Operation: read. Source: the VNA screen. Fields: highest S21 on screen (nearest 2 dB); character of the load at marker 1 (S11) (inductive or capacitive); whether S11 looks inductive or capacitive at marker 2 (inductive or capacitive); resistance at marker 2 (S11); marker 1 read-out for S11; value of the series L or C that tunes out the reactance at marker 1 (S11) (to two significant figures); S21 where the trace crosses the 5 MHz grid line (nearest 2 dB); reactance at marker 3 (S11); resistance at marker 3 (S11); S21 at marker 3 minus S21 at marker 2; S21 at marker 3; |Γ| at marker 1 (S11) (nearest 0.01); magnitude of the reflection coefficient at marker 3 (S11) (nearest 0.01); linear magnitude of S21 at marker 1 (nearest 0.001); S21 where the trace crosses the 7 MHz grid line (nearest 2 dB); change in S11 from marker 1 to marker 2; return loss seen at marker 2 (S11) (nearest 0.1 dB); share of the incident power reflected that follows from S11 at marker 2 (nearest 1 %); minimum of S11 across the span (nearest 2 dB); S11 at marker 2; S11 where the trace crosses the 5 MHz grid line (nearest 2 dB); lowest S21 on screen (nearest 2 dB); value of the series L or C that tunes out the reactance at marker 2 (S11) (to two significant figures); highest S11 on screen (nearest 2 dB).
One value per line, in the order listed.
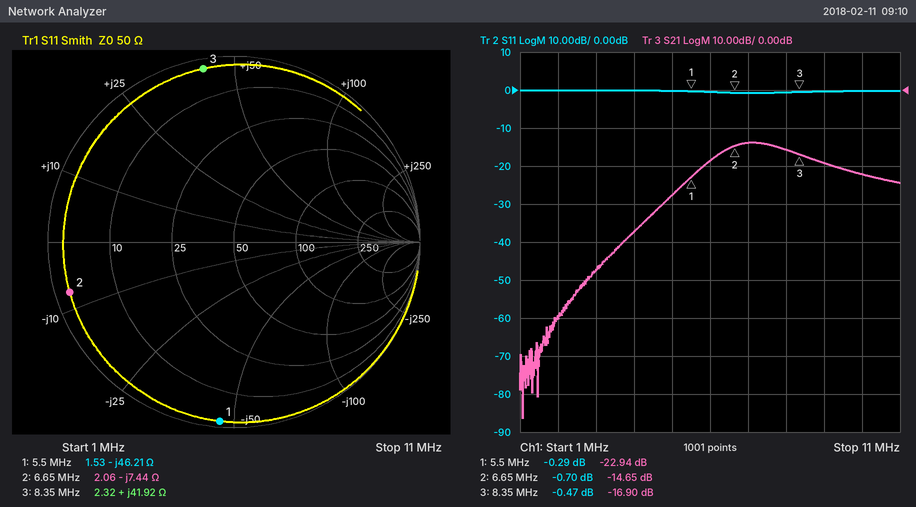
-14 dB
capacitive
capacitive
2.06 Ω
-0.29 dB
1.3 µH
-28 dB
+41.92 Ω
2.32 Ω
-2.25 dB
-16.90 dB
0.97
0.95
0.071
-14 dB
-0.41 dB
0.7 dB
85 %
0 dB
-0.70 dB
0 dB
-86 dB
180 nH
0 dB
